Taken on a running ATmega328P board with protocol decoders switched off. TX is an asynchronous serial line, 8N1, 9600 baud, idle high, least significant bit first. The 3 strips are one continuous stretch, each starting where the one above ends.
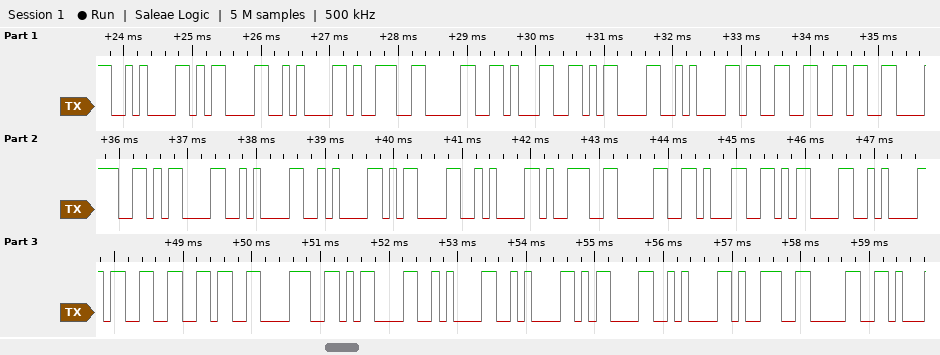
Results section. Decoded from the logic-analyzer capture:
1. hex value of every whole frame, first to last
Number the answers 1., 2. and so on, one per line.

1. 0A 0D 0A 39 30 31 0D 0A 33 36 38 0D 0A 0A 0D 0A 39 30 31 0D 0A 33 36 38 0D 0A 0A 0D 0A 39 30
